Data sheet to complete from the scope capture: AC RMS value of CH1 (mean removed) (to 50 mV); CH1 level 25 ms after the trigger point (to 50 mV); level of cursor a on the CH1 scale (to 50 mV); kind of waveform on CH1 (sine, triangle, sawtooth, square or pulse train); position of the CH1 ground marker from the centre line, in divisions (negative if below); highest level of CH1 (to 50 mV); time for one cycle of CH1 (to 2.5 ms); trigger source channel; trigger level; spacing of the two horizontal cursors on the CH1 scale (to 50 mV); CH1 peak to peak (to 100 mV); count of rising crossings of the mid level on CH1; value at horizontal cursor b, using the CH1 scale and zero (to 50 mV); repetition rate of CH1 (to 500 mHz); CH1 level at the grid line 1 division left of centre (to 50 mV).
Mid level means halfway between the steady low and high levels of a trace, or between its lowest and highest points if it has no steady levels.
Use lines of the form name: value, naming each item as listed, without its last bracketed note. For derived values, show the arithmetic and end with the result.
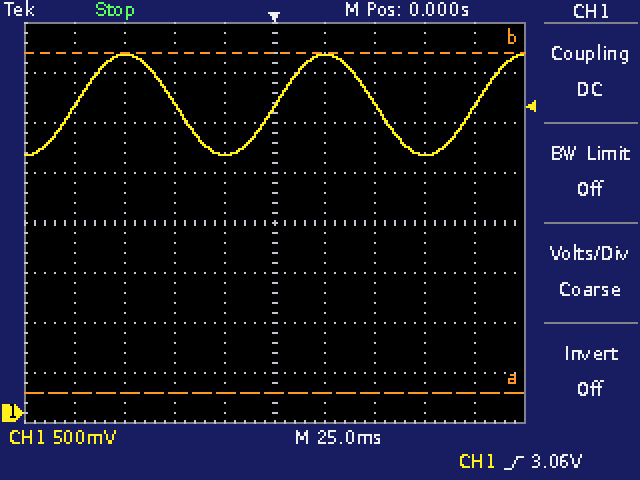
AC RMS value of CH1 (mean removed): 1.00 V / (2√2) ≈ 354 mV, so 350 mV to the nearest 50 mV
CH1 level 25 ms after the trigger point: 3.60 V
level of cursor a on the CH1 scale: 200 mV
kind of waveform on CH1: sine
position of the CH1 ground marker from the centre line, in divisions: -3.8 div
highest level of CH1: 3.60 V
time for one cycle of CH1: 100.0 ms
trigger source channel: CH1
trigger level: 3.06 V
spacing of the two horizontal cursors on the CH1 scale: 3.40 V
CH1 peak to peak: 1.00 V
count of rising crossings of the mid level on CH1: 3
value at horizontal cursor b, using the CH1 scale and zero: 3.60 V
repetition rate of CH1: 1 / 100.0 ms ≈ 10.0 Hz
CH1 level at the grid line 1 division left of centre: 2.60 V
